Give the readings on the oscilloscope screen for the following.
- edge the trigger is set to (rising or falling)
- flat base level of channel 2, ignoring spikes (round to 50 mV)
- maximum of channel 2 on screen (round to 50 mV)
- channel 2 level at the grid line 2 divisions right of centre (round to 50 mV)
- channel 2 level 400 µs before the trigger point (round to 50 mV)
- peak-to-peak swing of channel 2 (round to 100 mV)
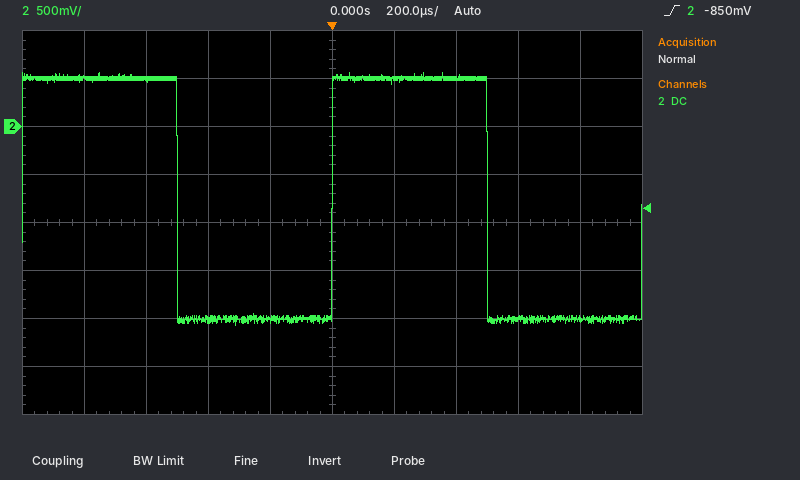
rising
-2.00 V
550 mV
500 mV
-2.00 V
2.60 V
